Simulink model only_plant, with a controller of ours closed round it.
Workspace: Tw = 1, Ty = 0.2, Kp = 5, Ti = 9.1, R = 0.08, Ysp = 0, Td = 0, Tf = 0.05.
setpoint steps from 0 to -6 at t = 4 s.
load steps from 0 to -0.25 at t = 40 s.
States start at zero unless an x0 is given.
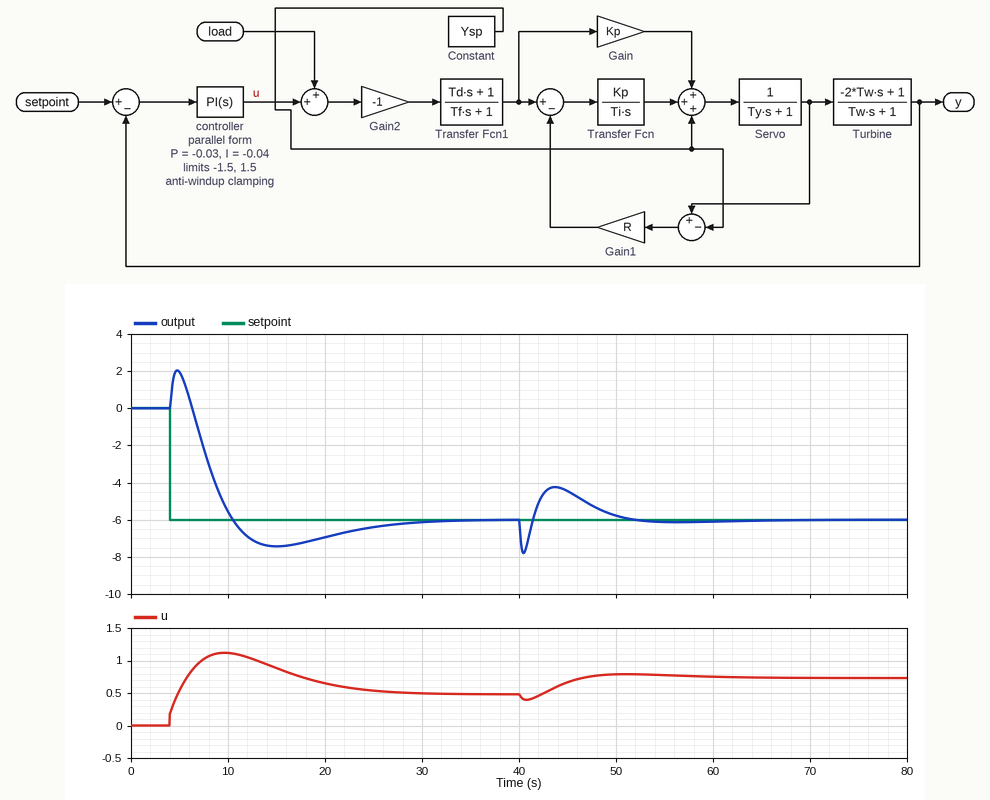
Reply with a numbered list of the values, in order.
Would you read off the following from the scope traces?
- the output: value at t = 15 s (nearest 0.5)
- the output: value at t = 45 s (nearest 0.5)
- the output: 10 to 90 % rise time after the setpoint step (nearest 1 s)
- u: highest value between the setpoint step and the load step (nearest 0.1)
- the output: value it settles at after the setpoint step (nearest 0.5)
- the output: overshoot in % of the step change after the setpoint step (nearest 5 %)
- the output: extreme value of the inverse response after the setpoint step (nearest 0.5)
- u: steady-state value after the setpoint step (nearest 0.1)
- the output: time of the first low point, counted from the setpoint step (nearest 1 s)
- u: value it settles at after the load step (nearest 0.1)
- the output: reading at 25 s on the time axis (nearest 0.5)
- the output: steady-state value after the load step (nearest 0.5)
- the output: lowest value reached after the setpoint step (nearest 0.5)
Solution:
1. -7.5
2. -4.5
3. 3 s
4. 1.1
5. -6.0
6. 25 %
7. 2.0
8. 0.5
9. 11 s
10. 0.7
11. -6.5
12. -6.0
13. -7.5
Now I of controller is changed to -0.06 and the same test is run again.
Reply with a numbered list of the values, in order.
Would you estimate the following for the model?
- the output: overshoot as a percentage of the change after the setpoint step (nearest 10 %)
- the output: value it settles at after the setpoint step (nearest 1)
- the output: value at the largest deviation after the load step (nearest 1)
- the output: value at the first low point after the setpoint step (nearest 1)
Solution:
1. 50 %
2. -6
3. -4
4. -9
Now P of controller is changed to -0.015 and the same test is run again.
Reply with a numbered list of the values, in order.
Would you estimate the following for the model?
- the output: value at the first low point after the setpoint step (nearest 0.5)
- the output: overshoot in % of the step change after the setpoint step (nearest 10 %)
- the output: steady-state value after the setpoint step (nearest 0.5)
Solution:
1. -8.0
2. 30 %
3. -6.0
